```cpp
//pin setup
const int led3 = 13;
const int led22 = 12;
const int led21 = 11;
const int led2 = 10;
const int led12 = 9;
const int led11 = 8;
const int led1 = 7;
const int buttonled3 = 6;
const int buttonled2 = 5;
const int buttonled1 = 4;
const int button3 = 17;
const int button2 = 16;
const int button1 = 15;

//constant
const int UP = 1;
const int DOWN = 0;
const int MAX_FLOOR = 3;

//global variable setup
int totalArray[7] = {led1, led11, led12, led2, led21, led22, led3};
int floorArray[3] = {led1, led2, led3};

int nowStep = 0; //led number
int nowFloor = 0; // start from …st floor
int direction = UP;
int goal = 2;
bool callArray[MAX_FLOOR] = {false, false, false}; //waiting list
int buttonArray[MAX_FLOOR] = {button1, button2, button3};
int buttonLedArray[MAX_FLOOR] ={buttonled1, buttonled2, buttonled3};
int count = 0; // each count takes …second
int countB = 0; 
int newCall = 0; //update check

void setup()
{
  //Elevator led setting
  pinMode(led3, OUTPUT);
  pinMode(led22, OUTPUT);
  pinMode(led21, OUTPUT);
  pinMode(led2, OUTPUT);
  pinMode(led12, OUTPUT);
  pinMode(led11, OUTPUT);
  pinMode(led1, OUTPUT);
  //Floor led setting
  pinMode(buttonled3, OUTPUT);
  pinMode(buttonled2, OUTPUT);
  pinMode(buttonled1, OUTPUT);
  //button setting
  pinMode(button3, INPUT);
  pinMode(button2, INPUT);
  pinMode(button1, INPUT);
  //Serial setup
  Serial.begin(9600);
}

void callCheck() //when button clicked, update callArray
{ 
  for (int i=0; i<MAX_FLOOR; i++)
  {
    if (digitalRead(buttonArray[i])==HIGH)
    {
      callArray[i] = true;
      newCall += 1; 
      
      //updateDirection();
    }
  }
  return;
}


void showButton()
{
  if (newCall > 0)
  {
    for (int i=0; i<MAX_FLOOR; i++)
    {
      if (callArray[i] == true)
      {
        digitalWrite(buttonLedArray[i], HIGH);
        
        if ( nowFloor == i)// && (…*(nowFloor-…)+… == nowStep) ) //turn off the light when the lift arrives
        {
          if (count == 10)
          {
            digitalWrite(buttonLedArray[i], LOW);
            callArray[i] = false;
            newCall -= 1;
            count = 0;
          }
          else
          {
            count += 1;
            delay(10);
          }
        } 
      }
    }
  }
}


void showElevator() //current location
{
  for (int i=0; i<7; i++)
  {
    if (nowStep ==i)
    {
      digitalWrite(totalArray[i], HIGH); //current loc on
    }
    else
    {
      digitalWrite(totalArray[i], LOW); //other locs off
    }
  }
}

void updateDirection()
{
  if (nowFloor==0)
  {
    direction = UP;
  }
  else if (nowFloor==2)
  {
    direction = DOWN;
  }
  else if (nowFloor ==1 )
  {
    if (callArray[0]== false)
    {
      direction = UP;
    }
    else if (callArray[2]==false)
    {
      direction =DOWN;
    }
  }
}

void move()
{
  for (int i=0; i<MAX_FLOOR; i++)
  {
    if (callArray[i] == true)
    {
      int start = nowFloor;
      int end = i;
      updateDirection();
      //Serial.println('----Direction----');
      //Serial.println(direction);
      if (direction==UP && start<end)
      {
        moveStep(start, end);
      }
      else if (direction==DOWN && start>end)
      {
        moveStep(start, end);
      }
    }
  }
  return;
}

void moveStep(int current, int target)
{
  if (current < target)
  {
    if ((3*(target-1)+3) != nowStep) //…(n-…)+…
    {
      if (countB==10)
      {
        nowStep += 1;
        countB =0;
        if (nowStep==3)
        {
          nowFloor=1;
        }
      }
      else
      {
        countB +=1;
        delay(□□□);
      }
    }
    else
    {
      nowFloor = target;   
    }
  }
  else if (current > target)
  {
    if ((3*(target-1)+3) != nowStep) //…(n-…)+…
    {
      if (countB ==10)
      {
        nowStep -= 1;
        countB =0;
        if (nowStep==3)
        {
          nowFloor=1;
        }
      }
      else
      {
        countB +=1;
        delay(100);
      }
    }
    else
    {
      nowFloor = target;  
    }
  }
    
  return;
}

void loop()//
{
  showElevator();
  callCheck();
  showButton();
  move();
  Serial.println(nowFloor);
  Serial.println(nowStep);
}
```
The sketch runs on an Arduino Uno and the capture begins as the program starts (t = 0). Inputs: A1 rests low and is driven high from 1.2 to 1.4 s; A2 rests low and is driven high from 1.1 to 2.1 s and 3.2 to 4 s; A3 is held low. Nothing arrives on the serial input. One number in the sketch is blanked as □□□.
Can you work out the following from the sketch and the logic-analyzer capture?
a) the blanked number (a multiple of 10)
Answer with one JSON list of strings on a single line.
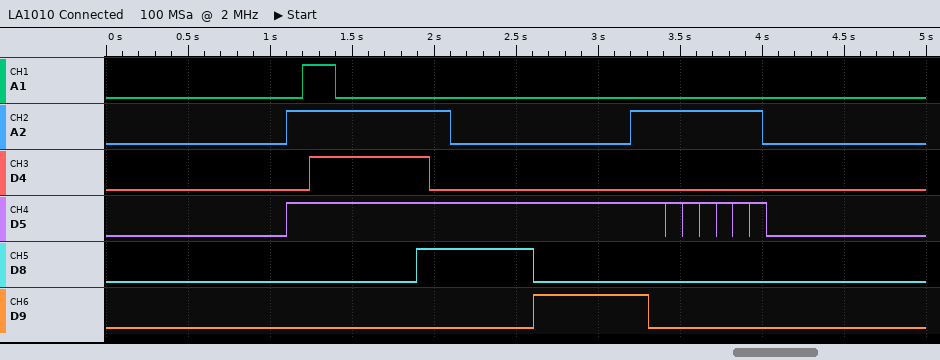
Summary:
["70"]
